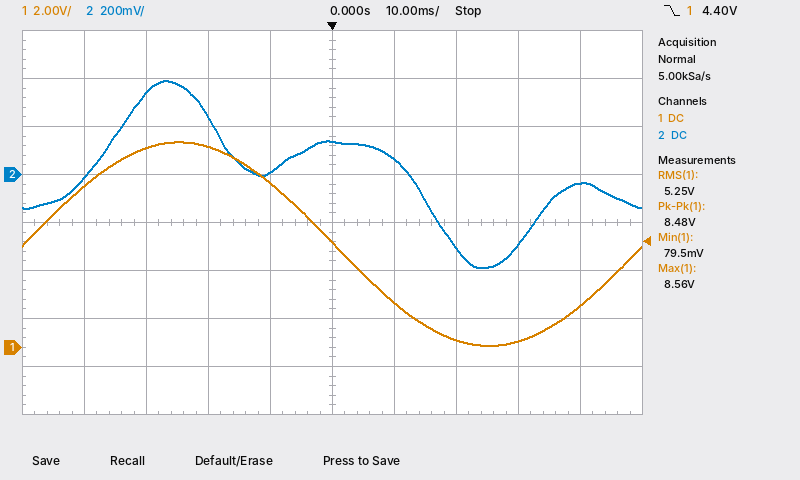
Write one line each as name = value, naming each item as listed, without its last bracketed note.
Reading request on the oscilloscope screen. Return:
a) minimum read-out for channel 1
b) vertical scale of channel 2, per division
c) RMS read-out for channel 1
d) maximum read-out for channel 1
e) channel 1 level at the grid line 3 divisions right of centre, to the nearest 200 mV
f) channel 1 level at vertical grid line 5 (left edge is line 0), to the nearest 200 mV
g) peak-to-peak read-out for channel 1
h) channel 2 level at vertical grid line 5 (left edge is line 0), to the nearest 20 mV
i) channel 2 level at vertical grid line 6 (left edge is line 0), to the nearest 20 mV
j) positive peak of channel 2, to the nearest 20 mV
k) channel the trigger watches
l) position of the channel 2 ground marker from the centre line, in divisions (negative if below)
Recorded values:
minimum read-out for channel 1 = 79.5 mV
vertical scale of channel 2, per division = 200 mV
RMS read-out for channel 1 = 5.25 V
maximum read-out for channel 1 = 8.56 V
channel 1 level at the grid line 3 divisions right of centre, to the nearest 200 mV = 200 mV
channel 1 level at vertical grid line 5 (left edge is line 0), to the nearest 200 mV = 4.4 V
peak-to-peak read-out for channel 1 = 8.48 V
channel 2 level at vertical grid line 5 (left edge is line 0), to the nearest 20 mV = 140 mV
channel 2 level at vertical grid line 6 (left edge is line 0), to the nearest 20 mV = 60 mV
positive peak of channel 2, to the nearest 20 mV = 400 mV
channel the trigger watches = channel 1
position of the channel 2 ground marker from the centre line, in divisions = +1.0 div
